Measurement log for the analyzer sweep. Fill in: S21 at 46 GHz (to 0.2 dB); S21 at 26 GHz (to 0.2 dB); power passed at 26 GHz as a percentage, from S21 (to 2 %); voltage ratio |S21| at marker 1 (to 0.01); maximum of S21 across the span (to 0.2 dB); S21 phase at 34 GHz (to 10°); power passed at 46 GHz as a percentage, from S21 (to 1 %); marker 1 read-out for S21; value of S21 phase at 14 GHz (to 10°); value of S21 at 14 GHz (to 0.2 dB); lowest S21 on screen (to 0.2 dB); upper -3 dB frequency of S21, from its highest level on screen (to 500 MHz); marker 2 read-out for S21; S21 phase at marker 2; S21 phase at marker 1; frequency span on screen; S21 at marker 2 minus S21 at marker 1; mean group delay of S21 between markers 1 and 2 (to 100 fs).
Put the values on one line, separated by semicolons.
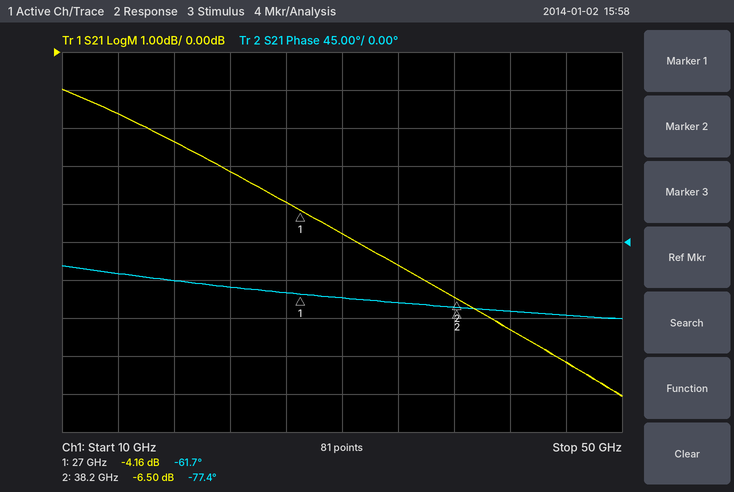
-8.2 dB; -4.0 dB; 40 %; 0.62; -1.0 dB; -70°; 15 %; -4.16 dB; -40°; -1.6 dB; -9.0 dB; 26.0 GHz; -6.50 dB; -77.4°; -61.7°; 40 GHz; -2.34 dB; 3.9 ps
